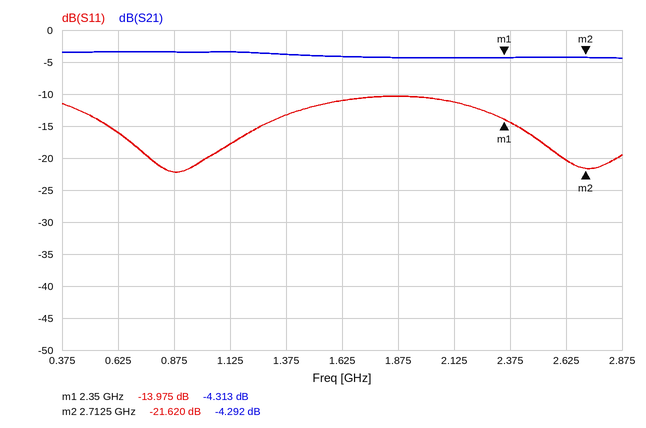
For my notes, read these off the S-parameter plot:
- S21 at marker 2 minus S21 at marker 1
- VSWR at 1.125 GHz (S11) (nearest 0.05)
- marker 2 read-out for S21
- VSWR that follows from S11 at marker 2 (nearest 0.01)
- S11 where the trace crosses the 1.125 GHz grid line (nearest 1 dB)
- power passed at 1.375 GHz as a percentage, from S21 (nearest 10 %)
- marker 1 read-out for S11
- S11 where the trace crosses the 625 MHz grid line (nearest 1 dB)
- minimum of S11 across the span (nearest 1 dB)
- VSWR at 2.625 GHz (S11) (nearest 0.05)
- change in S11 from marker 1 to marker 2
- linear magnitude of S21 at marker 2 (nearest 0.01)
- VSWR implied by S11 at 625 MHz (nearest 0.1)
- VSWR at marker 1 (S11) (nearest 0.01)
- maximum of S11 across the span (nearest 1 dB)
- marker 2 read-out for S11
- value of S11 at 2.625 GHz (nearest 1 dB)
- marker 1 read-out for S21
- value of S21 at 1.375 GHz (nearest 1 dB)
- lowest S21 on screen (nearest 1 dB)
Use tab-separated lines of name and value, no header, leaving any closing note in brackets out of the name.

S21 at marker 2 minus S21 at marker 1	0.021 dB
VSWR at 1.125 GHz (S11)	1.30
marker 2 read-out for S21	-4.292 dB
VSWR that follows from S11 at marker 2	1.18
S11 where the trace crosses the 1.125 GHz grid line	-18 dB
power passed at 1.375 GHz as a percentage, from S21	40 %
marker 1 read-out for S11	-13.975 dB
S11 where the trace crosses the 625 MHz grid line	-16 dB
minimum of S11 across the span	-22 dB
VSWR at 2.625 GHz (S11)	1.20
change in S11 from marker 1 to marker 2	-7.645 dB
linear magnitude of S21 at marker 2	0.61
VSWR implied by S11 at 625 MHz	1.4
VSWR at marker 1 (S11)	1.50
maximum of S11 across the span	-10 dB
marker 2 read-out for S11	-21.620 dB
value of S11 at 2.625 GHz	-20 dB
marker 1 read-out for S21	-4.313 dB
value of S21 at 1.375 GHz	-4 dB
lowest S21 on screen	-4 dB
